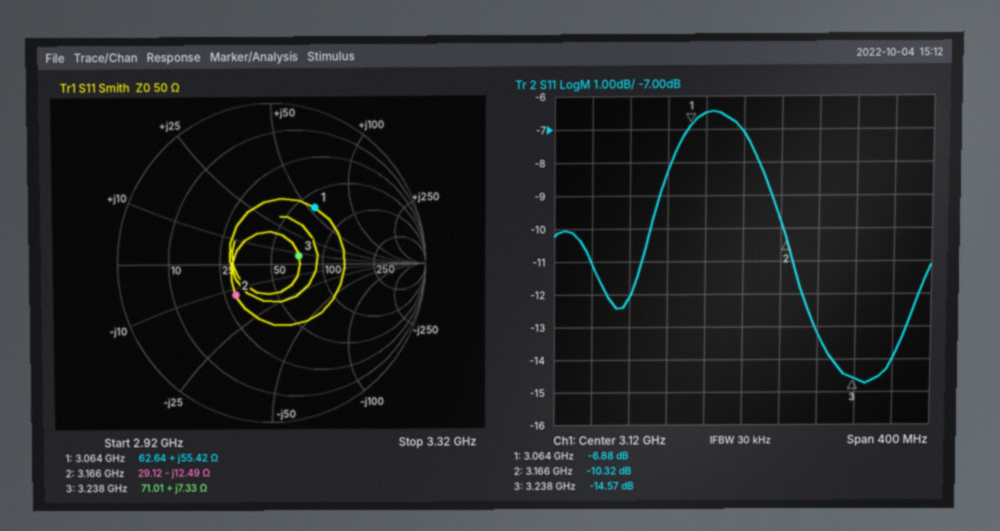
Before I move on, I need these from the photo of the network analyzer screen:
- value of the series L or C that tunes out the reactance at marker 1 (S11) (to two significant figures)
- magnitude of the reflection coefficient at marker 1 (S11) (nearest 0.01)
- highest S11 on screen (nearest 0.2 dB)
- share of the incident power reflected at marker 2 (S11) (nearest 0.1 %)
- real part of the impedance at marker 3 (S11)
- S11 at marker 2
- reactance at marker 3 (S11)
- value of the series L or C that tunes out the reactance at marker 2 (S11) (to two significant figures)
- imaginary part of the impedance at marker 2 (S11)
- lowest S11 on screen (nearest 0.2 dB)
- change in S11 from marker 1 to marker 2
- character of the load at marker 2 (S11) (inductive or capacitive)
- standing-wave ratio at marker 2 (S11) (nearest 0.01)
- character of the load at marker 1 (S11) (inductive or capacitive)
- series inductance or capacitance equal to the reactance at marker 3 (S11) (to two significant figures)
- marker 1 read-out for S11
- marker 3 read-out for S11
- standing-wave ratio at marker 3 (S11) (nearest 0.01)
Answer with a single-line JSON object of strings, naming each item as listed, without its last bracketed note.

{"value of the series L or C that tunes out the reactance at marker 1 (S11)": "940 fF", "magnitude of the reflection coefficient at marker 1 (S11)": "0.45", "highest S11 on screen": "-6.4 dB", "share of the incident power reflected at marker 2 (S11)": "9.3 %", "real part of the impedance at marker 3": "71.01 Ω", "S11 at marker 2": "-10.32 dB", "reactance at marker 3": "+7.33 Ω", "value of the series L or C that tunes out the reactance at marker 2 (S11)": "630 pH", "imaginary part of the impedance at marker 2": "-12.49 Ω", "lowest S11 on screen": "-14.8 dB", "change in S11 from marker 1 to marker 2": "-3.44 dB", "character of the load at marker 2 (S11)": "capacitive", "standing-wave ratio at marker 2 (S11)": "1.87", "character of the load at marker 1 (S11)": "inductive", "series inductance or capacitance equal to the reactance at marker 3 (S11)": "360 pH", "marker 1 read-out for S11": "-6.88 dB", "marker 3 read-out for S11": "-14.57 dB", "standing-wave ratio at marker 3 (S11)": "1.45"}
